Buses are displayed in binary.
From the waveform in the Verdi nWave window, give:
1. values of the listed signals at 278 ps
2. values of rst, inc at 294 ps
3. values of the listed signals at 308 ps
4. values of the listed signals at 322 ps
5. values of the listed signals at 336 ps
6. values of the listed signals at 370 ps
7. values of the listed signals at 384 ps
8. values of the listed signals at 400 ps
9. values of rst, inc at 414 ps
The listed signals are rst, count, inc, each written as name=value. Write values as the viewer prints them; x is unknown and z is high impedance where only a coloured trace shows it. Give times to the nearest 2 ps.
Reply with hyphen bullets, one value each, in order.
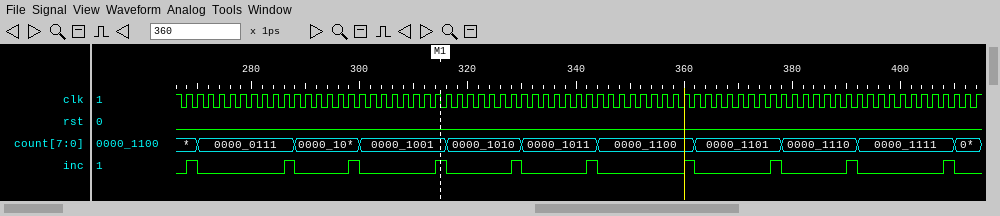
- rst=0, count=0000_0111, inc=0
- rst=0, inc=0
- rst=0, count=0000_1001, inc=0
- rst=0, count=0000_1010, inc=0
- rst=0, count=0000_1011, inc=0
- rst=0, count=0000_1101, inc=0
- rst=0, count=0000_1110, inc=0
- rst=0, count=0000_1111, inc=0
- rst=0, inc=0
